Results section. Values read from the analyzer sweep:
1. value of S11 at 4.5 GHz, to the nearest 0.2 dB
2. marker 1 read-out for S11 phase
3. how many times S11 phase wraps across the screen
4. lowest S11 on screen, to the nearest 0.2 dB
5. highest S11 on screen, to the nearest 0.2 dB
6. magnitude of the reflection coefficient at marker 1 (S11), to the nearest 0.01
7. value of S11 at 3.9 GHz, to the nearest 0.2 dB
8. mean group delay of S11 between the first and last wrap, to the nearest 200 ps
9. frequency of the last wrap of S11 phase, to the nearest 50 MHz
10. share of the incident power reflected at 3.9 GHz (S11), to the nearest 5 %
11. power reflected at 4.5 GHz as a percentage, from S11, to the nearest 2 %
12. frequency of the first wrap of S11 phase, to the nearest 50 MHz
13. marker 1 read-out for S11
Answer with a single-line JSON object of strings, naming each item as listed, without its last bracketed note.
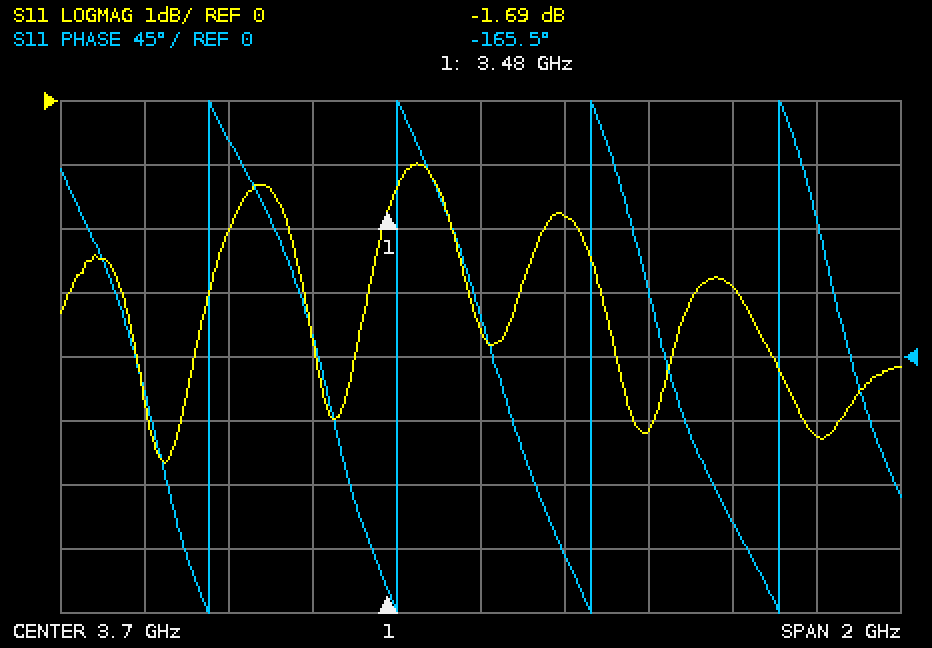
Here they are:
{"value of S11 at 4.5 GHz, to the nearest 0.2 dB": "-5.2 dB", "marker 1 read-out for S11 phase": "-165.5°", "how many times S11 phase wraps across the screen": "4", "lowest S11 on screen, to the nearest 0.2 dB": "-5.6 dB", "highest S11 on screen, to the nearest 0.2 dB": "-1.0 dB", "magnitude of the reflection coefficient at marker 1 (S11), to the nearest 0.01": "0.82", "value of S11 at 3.9 GHz, to the nearest 0.2 dB": "-1.8 dB", "mean group delay of S11 between the first and last wrap, to the nearest 200 ps": "2.2 ns", "frequency of the last wrap of S11 phase, to the nearest 50 MHz": "4.40 GHz", "share of the incident power reflected at 3.9 GHz (S11), to the nearest 5 %": "65 %", "power reflected at 4.5 GHz as a percentage, from S11, to the nearest 2 %": "30 %", "frequency of the first wrap of S11 phase, to the nearest 50 MHz": "3.05 GHz", "marker 1 read-out for S11": "-1.69 dB"}
